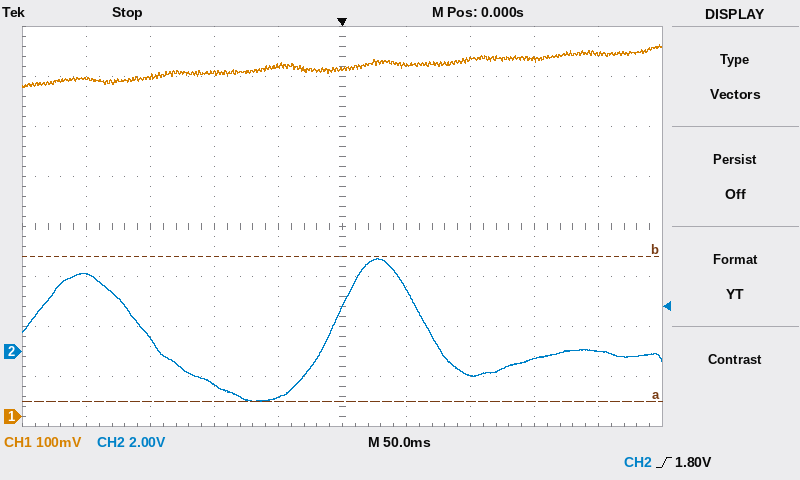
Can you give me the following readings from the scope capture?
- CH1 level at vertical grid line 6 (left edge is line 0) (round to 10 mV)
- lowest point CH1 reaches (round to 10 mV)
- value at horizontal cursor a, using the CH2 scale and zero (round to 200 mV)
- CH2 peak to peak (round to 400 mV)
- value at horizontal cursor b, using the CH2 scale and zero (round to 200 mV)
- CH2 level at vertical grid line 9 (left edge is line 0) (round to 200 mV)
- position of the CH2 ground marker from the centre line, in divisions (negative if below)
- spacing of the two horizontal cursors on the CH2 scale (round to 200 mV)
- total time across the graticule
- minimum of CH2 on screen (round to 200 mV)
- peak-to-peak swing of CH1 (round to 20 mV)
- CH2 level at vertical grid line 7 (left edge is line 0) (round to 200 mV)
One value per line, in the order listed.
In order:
700 mV
660 mV
-2.0 V
5.6 V
3.8 V
0.0 V
-2.5 div
5.8 V
500 ms
-2.0 V
80 mV
-1.0 V
